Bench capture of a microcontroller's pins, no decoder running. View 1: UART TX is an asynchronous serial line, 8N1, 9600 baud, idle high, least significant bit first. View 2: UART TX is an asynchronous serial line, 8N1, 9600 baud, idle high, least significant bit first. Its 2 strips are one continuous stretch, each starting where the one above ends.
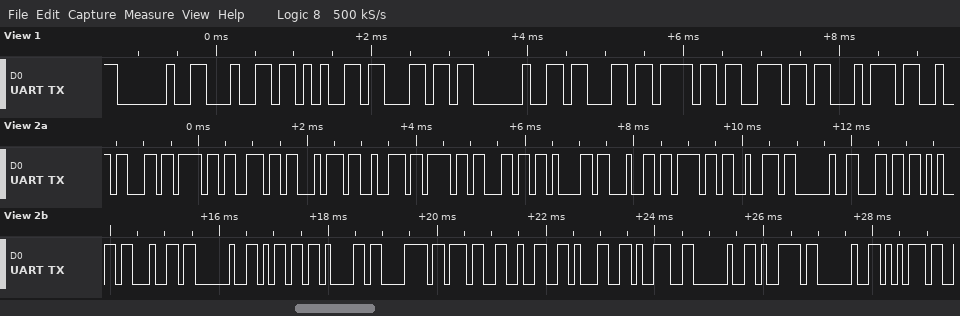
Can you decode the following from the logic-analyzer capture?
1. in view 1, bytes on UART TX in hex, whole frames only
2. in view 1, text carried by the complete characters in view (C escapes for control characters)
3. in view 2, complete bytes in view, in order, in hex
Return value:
20 64 65 6C 20 63 6F 6E 74
" del cont"
63 6F 6E 74 72 6F 6C 61 64 6F 72 20 6C 65 64 20 6D 61 78 37 32 31 39 20 79 20 75
